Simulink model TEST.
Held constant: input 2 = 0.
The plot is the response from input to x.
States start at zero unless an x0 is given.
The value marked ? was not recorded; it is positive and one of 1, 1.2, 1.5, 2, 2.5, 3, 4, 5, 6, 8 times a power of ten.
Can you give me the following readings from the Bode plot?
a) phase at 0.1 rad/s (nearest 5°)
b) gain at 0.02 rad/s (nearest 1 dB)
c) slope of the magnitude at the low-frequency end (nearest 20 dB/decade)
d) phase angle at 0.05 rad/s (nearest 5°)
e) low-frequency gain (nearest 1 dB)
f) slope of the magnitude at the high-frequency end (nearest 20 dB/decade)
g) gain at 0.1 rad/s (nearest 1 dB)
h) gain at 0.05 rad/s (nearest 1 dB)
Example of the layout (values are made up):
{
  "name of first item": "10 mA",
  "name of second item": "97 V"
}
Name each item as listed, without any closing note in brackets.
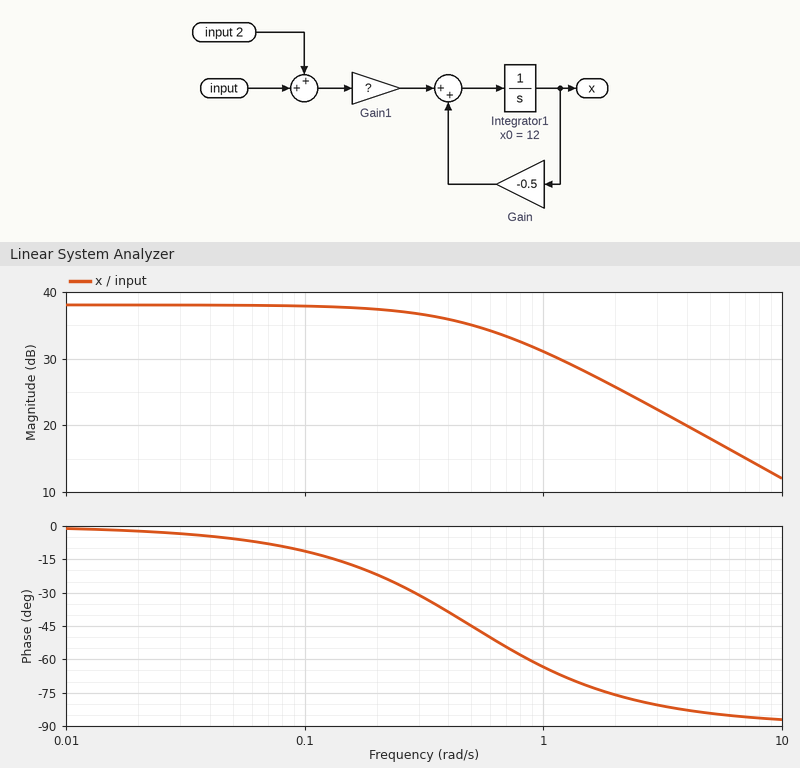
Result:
{
  "phase at 0.1 rad/s": "-10°",
  "gain at 0.02 rad/s": "38 dB",
  "slope of the magnitude at the low-frequency end": "0 dB/decade",
  "phase angle at 0.05 rad/s": "-5°",
  "low-frequency gain": "38 dB",
  "slope of the magnitude at the high-frequency end": "-20 dB/decade",
  "gain at 0.1 rad/s": "38 dB",
  "gain at 0.05 rad/s": "38 dB"
}
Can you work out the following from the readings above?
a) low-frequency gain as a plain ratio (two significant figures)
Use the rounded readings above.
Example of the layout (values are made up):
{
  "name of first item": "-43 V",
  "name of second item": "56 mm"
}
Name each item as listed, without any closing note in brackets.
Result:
{
  "low-frequency gain as a plain ratio": "79"
}
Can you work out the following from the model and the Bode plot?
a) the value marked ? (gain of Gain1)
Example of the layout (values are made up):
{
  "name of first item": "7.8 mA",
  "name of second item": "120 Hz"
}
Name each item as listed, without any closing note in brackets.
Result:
{
  "the value marked ?": "40"
}
